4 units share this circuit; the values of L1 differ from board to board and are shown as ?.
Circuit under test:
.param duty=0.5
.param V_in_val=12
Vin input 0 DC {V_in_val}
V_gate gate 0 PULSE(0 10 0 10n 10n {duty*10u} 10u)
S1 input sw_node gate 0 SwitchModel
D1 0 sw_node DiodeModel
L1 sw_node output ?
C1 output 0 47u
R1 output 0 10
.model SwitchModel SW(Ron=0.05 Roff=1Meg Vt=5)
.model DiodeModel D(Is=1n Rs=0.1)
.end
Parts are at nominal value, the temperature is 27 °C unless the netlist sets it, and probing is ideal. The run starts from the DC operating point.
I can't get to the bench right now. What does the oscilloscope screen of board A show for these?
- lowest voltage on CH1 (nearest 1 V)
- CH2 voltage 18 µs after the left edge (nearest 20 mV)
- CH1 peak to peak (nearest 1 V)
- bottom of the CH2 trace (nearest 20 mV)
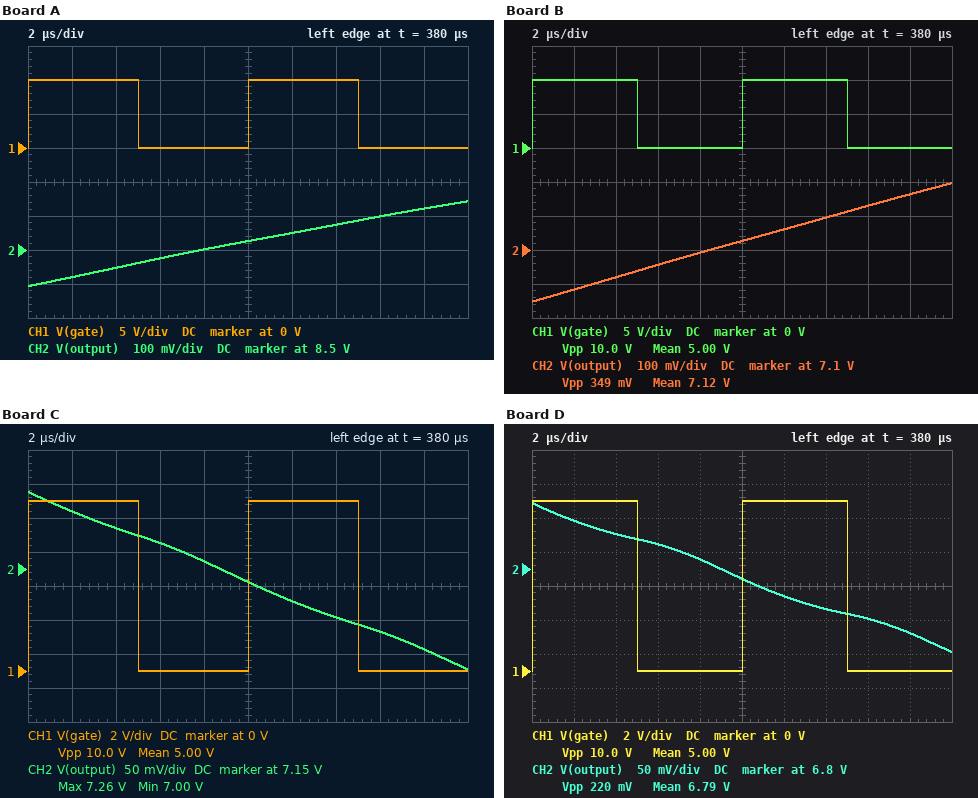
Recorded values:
0 V
8.62 V
10 V
8.40 V
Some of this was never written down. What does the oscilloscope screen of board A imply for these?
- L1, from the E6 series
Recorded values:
470 µH
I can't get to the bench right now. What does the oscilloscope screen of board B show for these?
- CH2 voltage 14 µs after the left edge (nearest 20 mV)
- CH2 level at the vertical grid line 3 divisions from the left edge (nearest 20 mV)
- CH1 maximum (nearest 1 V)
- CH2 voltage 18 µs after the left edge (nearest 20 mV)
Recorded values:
7.20 V
7.06 V
10 V
7.26 V
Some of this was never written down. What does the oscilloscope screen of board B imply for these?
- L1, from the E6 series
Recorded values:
680 µH
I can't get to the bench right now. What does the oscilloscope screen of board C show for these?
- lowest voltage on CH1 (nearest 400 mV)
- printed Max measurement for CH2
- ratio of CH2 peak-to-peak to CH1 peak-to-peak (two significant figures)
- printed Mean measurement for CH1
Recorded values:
0 V
7.26 V
0.026
5.00 V
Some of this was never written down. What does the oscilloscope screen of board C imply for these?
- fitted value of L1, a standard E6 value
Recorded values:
100 µH
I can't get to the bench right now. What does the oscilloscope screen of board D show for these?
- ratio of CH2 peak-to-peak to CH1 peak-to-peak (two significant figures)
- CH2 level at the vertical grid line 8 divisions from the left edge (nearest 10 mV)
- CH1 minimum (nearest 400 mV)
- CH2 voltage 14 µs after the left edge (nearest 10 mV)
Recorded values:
0.022
6.73 V
0 V
6.74 V
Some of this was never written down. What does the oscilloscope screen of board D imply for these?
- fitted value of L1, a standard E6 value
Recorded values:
68 µH
